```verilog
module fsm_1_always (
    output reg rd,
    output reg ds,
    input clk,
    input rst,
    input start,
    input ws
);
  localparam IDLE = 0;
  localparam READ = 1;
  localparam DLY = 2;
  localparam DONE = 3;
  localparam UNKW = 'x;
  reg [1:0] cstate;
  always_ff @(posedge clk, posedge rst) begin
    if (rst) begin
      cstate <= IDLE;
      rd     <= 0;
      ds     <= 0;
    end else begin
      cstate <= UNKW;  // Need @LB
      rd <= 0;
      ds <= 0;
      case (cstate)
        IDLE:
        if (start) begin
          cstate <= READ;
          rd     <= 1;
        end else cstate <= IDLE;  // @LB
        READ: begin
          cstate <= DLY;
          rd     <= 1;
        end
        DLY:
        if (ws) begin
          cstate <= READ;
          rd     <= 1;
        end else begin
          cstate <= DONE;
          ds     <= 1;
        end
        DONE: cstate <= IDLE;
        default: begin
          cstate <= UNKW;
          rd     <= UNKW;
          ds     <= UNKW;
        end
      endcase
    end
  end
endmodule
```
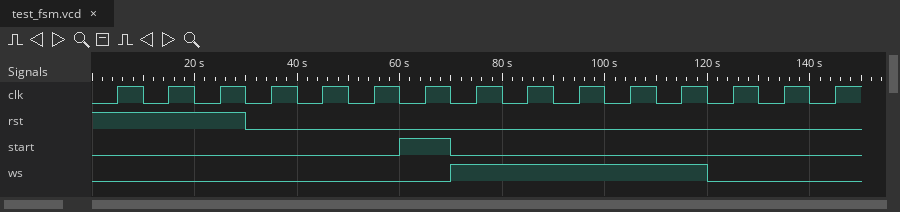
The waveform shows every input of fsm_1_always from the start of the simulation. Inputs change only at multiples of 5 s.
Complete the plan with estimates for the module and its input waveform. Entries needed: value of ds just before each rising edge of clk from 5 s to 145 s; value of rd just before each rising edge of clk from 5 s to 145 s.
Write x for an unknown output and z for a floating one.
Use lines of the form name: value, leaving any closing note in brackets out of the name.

value of ds just before each rising edge of clk from 5 s to 145 s: 0 0 0 0 0 0 0 0 0 0 0 0 0 1 0
value of rd just before each rising edge of clk from 5 s to 145 s: 0 0 0 0 0 0 0 1 1 1 1 1 1 0 0
